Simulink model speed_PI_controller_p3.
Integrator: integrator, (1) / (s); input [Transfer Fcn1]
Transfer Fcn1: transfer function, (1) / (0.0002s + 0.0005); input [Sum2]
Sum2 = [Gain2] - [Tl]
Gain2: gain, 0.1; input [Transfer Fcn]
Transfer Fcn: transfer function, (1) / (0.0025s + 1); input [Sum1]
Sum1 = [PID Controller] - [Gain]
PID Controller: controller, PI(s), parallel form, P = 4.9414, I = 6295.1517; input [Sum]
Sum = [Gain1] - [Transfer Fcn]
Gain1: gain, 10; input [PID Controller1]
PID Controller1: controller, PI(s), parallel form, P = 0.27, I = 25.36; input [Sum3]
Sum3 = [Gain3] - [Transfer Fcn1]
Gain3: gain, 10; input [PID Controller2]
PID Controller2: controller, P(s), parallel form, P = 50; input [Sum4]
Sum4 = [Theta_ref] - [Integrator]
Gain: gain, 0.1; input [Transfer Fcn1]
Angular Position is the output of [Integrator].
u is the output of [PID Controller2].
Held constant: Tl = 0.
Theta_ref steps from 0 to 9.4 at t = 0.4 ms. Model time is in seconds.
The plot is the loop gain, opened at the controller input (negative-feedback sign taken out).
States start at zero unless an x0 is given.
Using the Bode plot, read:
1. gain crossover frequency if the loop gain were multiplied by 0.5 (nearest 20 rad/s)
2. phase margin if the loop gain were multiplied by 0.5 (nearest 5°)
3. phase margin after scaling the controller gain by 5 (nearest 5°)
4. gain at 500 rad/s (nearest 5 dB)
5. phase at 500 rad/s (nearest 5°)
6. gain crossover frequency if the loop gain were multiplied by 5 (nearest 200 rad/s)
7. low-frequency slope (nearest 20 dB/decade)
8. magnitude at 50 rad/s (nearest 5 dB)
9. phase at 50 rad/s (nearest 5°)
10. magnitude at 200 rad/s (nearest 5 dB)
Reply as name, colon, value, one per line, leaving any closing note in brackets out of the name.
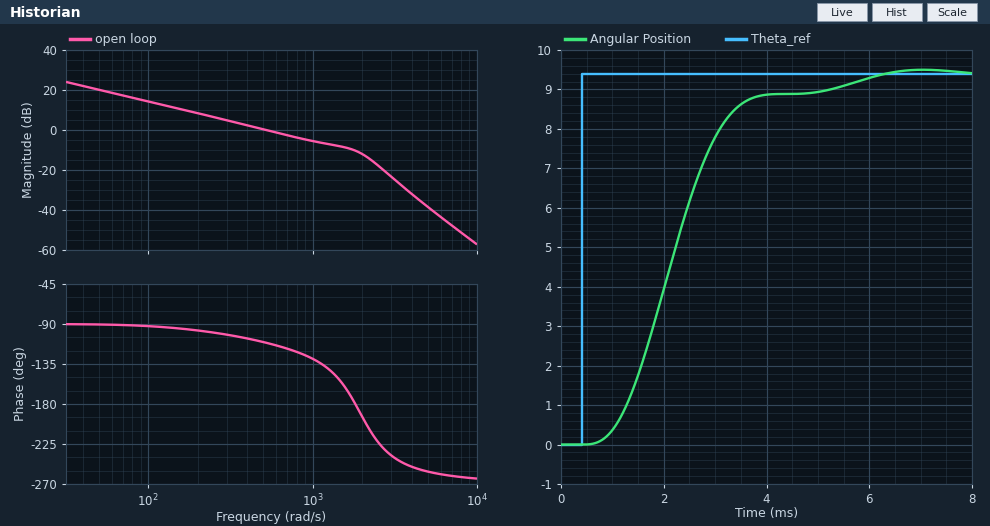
gain crossover frequency if the loop gain were multiplied by 0.5: 260 rad/s
phase margin if the loop gain were multiplied by 0.5: 80°
phase margin after scaling the controller gain by 5: -25°
gain at 500 rad/s: 0 dB
phase at 500 rad/s: -110°
gain crossover frequency if the loop gain were multiplied by 5: 2200 rad/s
low-frequency slope: -20 dB/decade
magnitude at 50 rad/s: 20 dB
phase at 50 rad/s: -90°
magnitude at 200 rad/s: 10 dB
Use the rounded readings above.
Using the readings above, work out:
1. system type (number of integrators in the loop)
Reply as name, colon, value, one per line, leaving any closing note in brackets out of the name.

system type: 1
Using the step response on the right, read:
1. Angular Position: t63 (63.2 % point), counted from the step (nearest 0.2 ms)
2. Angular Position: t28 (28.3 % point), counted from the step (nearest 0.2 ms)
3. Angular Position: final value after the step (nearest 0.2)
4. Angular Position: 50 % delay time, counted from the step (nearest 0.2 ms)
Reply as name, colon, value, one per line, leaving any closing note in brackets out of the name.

Angular Position: t63 (63.2 % point), counted from the step: 2.0 ms
Angular Position: t28 (28.3 % point), counted from the step: 1.4 ms
Angular Position: final value after the step: 9.4
Angular Position: 50 % delay time, counted from the step: 1.8 ms
